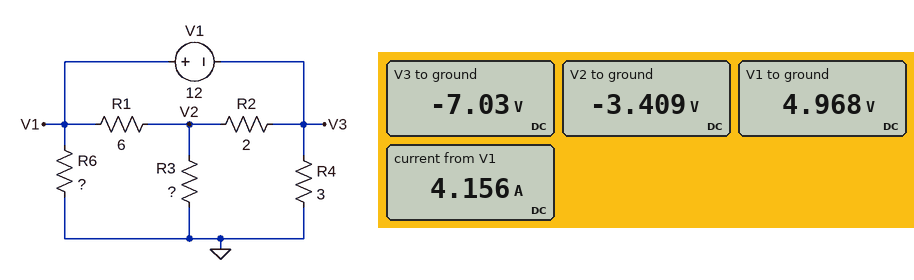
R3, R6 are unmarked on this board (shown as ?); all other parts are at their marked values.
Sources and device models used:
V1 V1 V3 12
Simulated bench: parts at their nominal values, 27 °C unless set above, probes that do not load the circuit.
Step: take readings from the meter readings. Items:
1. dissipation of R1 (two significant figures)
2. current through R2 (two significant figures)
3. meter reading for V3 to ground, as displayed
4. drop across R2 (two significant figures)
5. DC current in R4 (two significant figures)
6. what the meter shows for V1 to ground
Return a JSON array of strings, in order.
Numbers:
["12 W", "1.8 A", "-7.03 V", "3.6 V", "2.3 A", "4.968 V"]
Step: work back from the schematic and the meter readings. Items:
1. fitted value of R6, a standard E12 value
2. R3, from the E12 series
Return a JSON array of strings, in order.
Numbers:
["1.8 Ω", "8.2 Ω"]
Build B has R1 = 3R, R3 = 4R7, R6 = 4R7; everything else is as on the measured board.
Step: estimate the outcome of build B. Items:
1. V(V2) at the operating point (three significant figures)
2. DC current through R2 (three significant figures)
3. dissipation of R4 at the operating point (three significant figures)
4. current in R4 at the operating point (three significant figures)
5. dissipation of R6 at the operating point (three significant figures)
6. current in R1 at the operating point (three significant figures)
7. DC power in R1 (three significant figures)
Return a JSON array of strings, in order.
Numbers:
["75.8 mV", "2.39 A", "7.38 W", "1.57 A", "11.3 W", "2.41 A", "17.4 W"]
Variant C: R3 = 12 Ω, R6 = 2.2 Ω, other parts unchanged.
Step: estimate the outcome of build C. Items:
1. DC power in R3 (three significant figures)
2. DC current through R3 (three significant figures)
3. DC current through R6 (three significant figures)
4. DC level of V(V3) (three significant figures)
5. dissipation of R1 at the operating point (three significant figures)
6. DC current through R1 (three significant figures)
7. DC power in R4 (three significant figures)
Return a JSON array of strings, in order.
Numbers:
["847 mW", "266 mA", "2.46 A", "-6.59 V", "12.3 W", "1.43 A", "14.5 W"]
